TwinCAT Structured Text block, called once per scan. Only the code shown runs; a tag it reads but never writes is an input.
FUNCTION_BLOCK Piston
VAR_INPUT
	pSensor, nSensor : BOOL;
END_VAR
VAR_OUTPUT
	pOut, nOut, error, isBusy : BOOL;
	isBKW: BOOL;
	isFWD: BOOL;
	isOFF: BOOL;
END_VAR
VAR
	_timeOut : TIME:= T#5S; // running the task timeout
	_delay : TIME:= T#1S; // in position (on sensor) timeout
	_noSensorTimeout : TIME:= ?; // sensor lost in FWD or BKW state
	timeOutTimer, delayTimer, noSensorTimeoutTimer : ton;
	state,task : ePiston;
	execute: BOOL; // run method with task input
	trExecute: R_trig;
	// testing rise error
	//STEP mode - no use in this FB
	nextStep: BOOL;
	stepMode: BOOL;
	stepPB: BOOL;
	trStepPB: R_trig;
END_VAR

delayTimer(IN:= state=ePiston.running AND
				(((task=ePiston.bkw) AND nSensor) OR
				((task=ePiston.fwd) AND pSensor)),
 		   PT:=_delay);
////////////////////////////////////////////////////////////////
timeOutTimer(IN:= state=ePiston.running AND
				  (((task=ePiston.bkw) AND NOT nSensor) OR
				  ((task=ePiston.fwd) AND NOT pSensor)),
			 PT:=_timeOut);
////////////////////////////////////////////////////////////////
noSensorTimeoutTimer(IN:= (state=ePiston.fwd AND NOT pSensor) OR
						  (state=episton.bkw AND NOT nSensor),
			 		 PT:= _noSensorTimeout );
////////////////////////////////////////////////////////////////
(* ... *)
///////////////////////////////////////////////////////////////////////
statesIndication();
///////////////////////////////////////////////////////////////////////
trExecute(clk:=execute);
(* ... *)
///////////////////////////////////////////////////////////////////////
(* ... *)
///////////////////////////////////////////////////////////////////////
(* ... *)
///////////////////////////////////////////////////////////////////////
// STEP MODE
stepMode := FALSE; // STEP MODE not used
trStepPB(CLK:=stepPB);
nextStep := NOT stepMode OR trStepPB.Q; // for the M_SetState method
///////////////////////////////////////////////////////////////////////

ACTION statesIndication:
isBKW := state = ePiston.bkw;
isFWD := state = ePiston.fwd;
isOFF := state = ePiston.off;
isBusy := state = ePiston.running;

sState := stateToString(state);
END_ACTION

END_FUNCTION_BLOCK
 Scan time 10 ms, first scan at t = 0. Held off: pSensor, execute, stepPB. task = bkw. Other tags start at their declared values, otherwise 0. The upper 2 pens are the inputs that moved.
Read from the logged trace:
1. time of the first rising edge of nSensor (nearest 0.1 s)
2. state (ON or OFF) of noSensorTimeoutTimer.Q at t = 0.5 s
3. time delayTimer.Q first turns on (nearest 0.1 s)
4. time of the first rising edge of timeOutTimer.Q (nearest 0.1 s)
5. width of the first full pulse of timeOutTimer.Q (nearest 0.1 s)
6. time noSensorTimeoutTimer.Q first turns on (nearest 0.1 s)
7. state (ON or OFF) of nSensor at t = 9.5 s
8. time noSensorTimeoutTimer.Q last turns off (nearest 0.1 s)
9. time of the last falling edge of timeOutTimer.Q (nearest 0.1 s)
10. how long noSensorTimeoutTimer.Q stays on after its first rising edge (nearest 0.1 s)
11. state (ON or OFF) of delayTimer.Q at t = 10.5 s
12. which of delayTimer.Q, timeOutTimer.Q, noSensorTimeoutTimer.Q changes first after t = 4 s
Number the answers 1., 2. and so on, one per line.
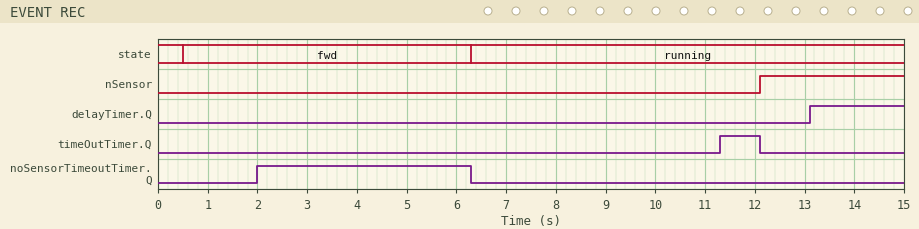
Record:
1. 12.1 s
2. OFF
3. 13.1 s
4. 11.3 s
5. 0.8 s
6. 2.0 s
7. OFF
8. 6.3 s
9. 12.1 s
10. 4.3 s
11. OFF
12. noSensorTimeoutTimer.Q
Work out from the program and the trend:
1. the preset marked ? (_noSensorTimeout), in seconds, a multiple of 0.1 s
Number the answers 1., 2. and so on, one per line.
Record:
1. 1.5 s
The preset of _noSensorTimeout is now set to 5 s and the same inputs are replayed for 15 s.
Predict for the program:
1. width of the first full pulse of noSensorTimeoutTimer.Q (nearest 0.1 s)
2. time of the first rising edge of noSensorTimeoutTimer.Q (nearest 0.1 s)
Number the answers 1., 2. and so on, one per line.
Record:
1. 0.8 s
2. 5.5 s
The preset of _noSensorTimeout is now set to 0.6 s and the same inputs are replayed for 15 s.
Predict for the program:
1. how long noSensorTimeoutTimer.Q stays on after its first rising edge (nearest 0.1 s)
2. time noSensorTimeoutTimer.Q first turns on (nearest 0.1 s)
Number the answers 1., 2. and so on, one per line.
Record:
1. 5.2 s
2. 1.1 s
